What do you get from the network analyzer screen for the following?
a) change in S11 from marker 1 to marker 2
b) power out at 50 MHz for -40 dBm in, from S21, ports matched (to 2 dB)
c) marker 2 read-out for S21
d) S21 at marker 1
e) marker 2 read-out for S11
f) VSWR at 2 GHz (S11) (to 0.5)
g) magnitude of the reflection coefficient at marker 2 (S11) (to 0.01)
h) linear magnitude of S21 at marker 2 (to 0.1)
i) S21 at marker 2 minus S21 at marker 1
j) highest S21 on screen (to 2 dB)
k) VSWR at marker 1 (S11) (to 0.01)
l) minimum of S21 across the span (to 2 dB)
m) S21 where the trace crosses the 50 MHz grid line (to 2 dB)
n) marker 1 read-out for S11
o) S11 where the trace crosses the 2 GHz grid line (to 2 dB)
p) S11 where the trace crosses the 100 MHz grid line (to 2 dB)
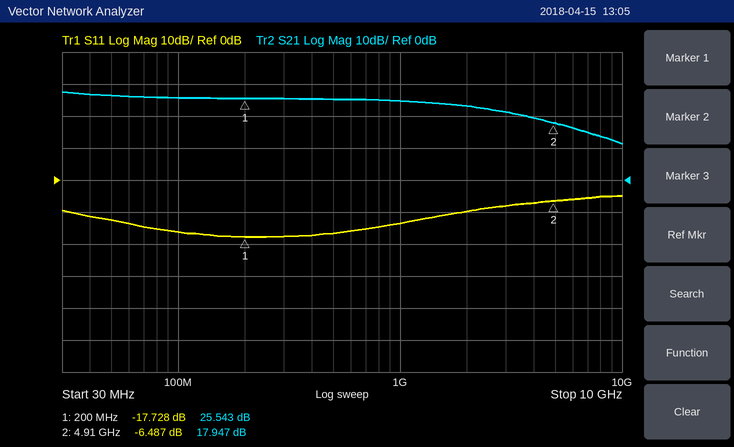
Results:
11.241 dB
-14 dBm
17.947 dB
25.543 dB
-6.487 dB
2.0
0.47
7.9
-7.596 dB
28 dB
1.30
12 dB
26 dB
-17.728 dB
-10 dB
-16 dB
